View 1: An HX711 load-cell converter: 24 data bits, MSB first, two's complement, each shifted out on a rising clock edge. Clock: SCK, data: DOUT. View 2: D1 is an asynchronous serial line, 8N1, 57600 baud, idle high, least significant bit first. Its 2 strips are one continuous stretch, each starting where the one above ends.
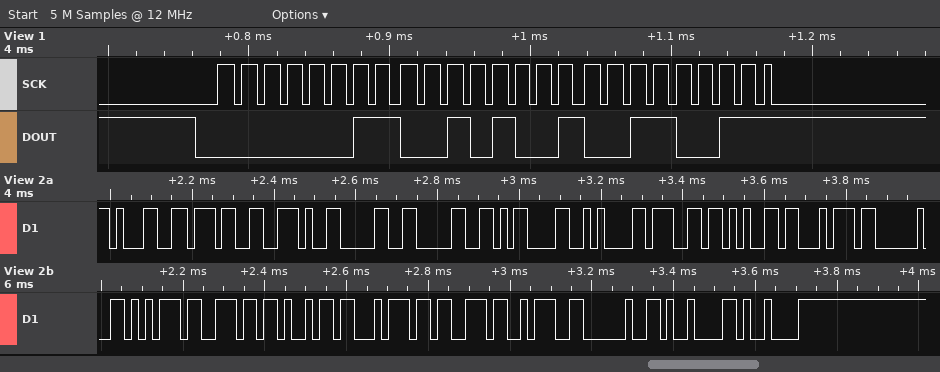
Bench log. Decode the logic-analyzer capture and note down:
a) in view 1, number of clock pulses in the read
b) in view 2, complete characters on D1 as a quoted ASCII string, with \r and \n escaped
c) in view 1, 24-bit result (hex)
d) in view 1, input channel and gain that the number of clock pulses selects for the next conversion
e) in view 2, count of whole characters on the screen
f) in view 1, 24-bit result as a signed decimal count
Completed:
25
"17.00\r\nget units: \t\t"
0x032933
channel A, gain 128
20
207155
